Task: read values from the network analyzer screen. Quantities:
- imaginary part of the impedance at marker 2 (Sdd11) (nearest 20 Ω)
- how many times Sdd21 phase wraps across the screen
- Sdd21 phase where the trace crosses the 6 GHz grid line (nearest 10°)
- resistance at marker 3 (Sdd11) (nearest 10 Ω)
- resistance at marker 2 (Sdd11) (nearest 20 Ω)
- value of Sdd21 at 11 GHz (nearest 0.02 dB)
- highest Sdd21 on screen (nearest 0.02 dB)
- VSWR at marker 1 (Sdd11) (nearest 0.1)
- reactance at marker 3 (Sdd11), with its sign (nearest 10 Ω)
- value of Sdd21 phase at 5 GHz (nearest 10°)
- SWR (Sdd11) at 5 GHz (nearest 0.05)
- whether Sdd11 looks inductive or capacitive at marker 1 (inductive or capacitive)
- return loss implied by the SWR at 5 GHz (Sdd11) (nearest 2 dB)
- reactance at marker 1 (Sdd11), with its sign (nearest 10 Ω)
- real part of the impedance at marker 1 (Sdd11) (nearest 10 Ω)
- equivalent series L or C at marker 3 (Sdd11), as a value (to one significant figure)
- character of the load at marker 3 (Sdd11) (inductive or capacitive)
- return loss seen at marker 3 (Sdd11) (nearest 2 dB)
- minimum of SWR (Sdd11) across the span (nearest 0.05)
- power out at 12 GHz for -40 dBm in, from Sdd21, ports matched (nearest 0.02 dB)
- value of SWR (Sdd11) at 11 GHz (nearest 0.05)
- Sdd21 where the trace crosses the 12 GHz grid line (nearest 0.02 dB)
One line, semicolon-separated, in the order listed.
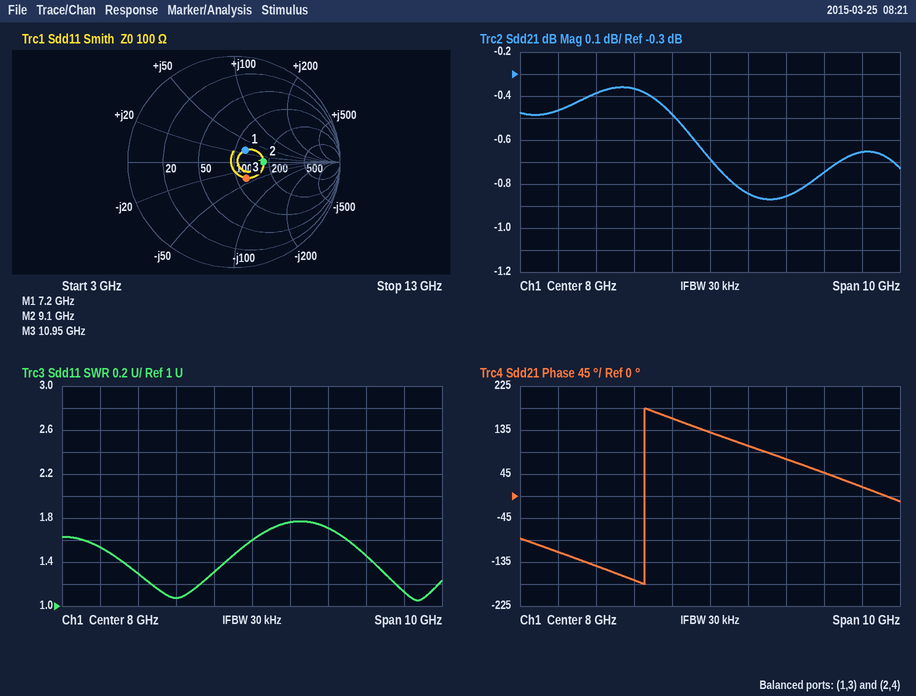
0 Ω; 1; -170°; 120 Ω; 180 Ω; -0.74 dB; -0.36 dB; 1.4; -40 Ω; -140°; 1.30; inductive; 18 dB; +30 Ω; 120 Ω; 400 fF; capacitive; 14 dB; 1.05; -40.66 dBm; 1.45; -0.66 dB
